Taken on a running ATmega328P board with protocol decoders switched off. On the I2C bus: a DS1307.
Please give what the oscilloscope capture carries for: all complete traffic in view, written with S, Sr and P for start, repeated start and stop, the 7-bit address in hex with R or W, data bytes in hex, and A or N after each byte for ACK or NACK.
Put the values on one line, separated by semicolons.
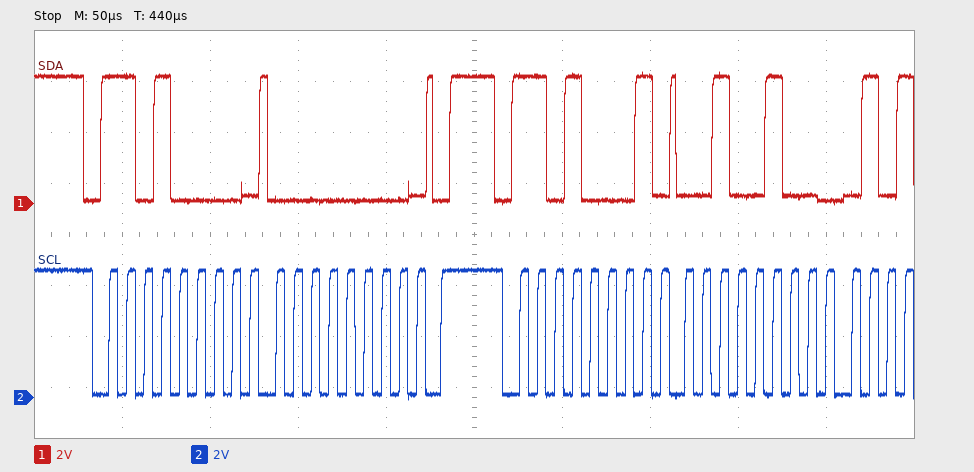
S 68W A 00 A P S 68R A 24 A
